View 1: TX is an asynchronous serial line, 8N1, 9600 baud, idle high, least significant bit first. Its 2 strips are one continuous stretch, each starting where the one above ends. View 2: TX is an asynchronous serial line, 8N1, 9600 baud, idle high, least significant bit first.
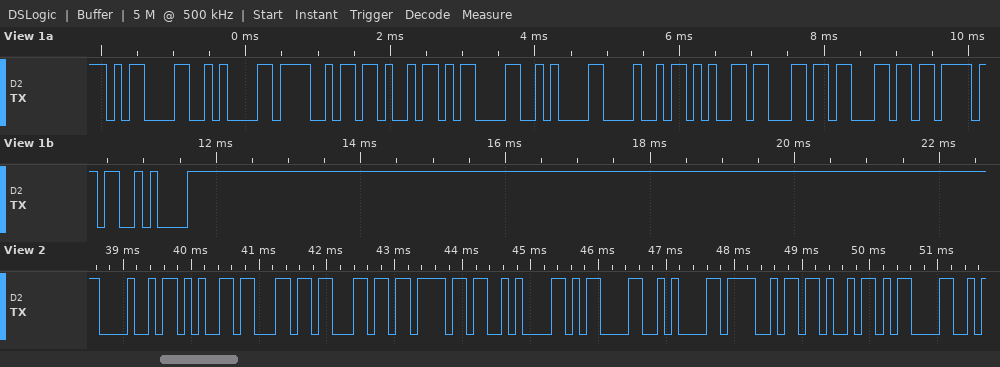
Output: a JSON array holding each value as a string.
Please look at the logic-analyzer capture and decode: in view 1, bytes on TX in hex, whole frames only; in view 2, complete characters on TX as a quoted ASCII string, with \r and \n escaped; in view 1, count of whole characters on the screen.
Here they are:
["0x0D 0x0A 0x4F 0x4B 0x0D 0x0A 0x48 0x65 0x6C 0x6C 0x6F 0x0A", "\"Hello\\n\\r\\nOK\\r\"", "12"]
